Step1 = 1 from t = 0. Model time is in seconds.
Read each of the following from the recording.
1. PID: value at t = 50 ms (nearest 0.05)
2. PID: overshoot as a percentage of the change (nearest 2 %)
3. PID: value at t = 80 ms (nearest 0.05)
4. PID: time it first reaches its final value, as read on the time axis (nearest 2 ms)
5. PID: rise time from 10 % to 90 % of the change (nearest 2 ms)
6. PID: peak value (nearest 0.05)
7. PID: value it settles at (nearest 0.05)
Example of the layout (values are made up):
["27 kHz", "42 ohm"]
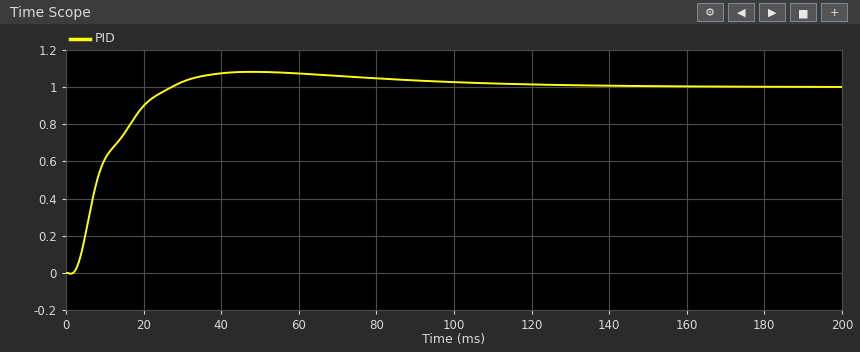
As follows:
["1.10", "8 %", "1.05", "28 ms", "16 ms", "1.10", "1.00"]
